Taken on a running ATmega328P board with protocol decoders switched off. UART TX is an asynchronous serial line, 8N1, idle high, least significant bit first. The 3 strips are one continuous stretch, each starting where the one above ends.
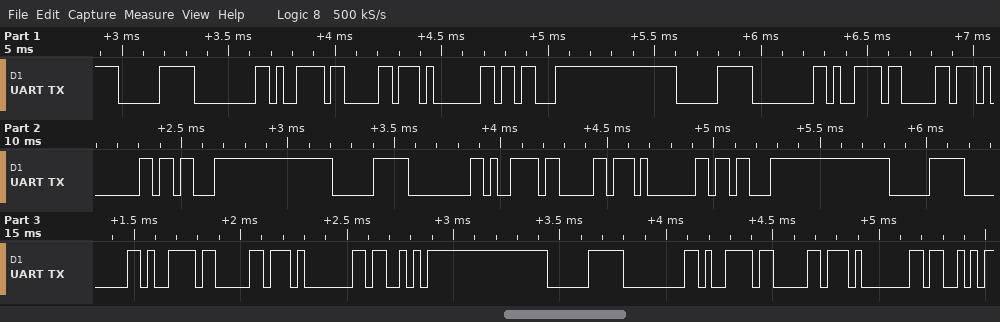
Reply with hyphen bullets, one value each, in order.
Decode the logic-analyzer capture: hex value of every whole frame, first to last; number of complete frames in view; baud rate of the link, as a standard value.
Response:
- E0 00 79 B0 01 1B E0 00 79 B0 01 1B E0 00 79 B0 01 1B E0 00 79 B0 01 53 E0 00 79 B0 01 53
- 30
- 31250 baud
